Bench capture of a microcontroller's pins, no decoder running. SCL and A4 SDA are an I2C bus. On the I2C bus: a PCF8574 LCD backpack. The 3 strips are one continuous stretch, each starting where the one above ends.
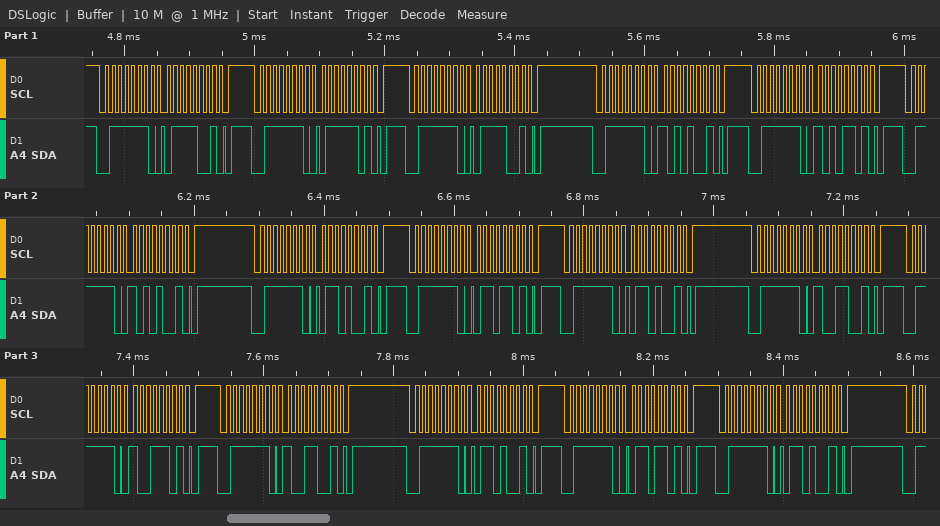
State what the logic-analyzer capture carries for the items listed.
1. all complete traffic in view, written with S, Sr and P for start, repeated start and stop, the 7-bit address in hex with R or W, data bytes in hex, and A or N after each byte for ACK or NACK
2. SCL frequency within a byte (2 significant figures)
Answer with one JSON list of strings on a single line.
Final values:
["S 3FW A 79 A P S 3FW A 7D A P S 3FW A 79 A P S 3FW A A9 A P S 3FW A AD A P S 3FW A A9 A P S 3FW A 69 A P S 3FW A 6D A P S 3FW A 69 A P S 3FW A 99 A P S 3FW A 9D A P S 3FW A 99 A P S 3FW A 69 A P S 3FW A 6D A P S 3FW A 69 A P", "100 kHz"]
